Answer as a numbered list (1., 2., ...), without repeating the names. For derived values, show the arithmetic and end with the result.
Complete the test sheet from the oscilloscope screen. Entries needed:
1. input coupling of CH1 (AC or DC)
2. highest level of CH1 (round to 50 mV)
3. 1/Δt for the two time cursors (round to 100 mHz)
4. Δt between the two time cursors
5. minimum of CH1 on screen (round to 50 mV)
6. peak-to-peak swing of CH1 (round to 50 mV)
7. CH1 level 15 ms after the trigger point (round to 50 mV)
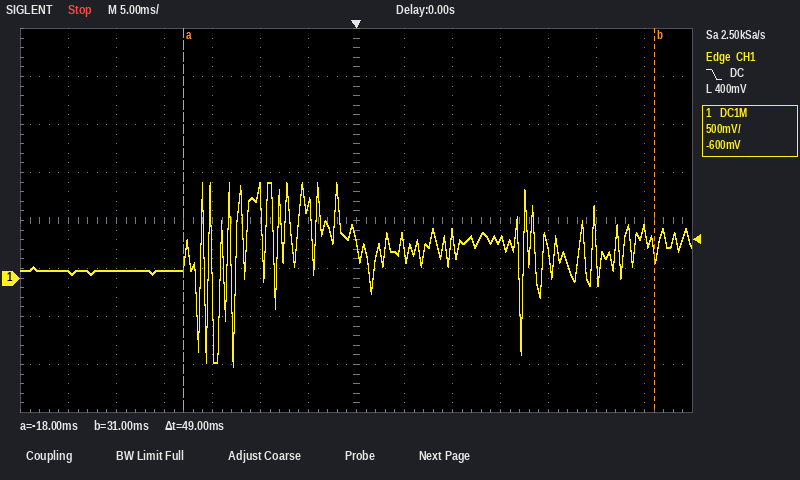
1. DC
2. 1.00 V
3. 1 / 49 ms ≈ 20.4 Hz
4. 49 ms
5. -900 mV
6. 1.00 V − (-900 mV) = 1.90 V
7. 400 mV
